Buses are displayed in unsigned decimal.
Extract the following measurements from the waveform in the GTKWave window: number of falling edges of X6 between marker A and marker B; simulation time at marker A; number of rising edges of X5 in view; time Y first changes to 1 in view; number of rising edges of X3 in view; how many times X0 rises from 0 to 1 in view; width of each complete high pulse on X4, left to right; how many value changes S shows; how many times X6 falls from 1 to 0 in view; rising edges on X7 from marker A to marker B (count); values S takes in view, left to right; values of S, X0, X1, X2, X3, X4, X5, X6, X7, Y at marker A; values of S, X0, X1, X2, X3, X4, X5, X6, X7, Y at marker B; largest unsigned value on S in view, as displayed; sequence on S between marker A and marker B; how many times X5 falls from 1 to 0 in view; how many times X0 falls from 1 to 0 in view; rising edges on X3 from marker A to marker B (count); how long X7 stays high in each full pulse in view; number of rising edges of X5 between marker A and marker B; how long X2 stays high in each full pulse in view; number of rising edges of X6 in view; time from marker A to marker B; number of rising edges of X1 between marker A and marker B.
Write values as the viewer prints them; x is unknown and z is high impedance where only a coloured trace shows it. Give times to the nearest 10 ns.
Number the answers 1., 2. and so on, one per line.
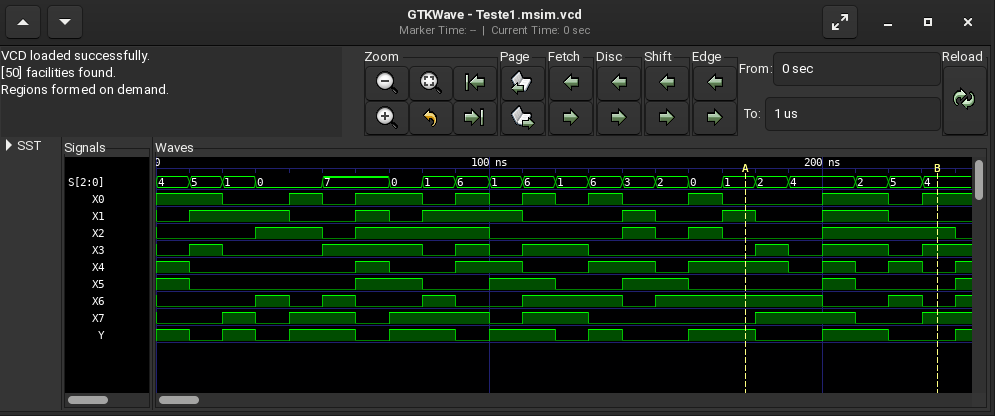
1. 2
2. 180 ns
3. 5
4. 20 ns
5. 7
6. 8
7. 10 ns, 20 ns, 20 ns, 30 ns, 10 ns, 10 ns
8. 20
9. 6
10. 2
11. 4, 5, 1, 0, 7, 0, 1, 6, 1, 6, 1, 6, 3, 2, 0, 1, 2, 4, 2, 5, 4
12. S=1, X0=0, X1=1, X2=0, X3=0, X4=1, X5=0, X6=1, X7=0, Y=1
13. S=4, X0=1, X1=0, X2=1, X3=1, X4=0, X5=0, X6=0, X7=1, Y=0
14. 7
15. 1, 2, 4, 2, 5, 4
16. 5
17. 8
18. 3
19. 10 ns, 20 ns, 30 ns, 20 ns, 30 ns
20. 1
21. 20 ns, 40 ns, 10 ns, 10 ns, 40 ns
22. 7
23. 60 ns
24. 1
